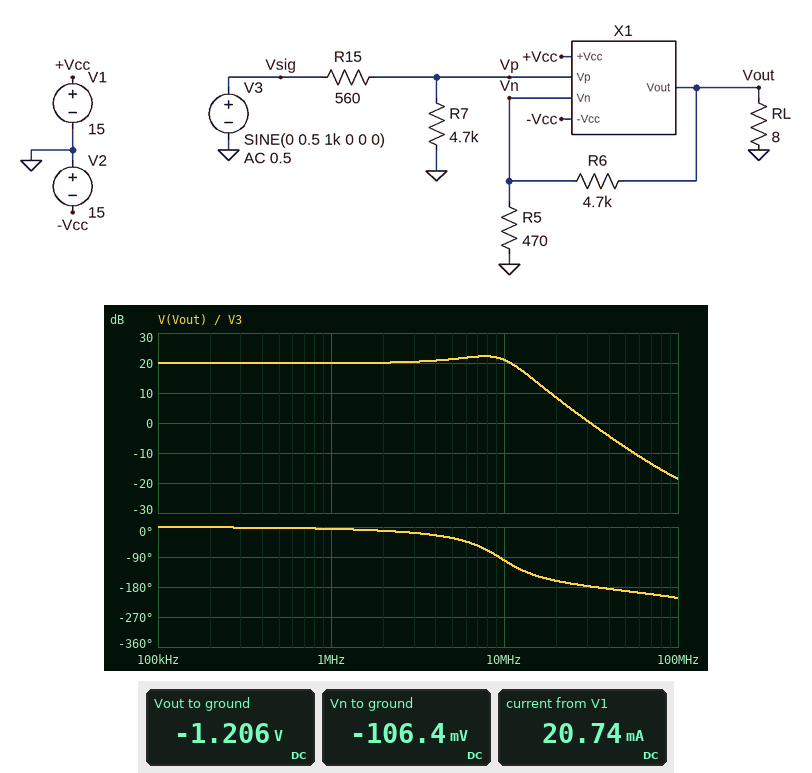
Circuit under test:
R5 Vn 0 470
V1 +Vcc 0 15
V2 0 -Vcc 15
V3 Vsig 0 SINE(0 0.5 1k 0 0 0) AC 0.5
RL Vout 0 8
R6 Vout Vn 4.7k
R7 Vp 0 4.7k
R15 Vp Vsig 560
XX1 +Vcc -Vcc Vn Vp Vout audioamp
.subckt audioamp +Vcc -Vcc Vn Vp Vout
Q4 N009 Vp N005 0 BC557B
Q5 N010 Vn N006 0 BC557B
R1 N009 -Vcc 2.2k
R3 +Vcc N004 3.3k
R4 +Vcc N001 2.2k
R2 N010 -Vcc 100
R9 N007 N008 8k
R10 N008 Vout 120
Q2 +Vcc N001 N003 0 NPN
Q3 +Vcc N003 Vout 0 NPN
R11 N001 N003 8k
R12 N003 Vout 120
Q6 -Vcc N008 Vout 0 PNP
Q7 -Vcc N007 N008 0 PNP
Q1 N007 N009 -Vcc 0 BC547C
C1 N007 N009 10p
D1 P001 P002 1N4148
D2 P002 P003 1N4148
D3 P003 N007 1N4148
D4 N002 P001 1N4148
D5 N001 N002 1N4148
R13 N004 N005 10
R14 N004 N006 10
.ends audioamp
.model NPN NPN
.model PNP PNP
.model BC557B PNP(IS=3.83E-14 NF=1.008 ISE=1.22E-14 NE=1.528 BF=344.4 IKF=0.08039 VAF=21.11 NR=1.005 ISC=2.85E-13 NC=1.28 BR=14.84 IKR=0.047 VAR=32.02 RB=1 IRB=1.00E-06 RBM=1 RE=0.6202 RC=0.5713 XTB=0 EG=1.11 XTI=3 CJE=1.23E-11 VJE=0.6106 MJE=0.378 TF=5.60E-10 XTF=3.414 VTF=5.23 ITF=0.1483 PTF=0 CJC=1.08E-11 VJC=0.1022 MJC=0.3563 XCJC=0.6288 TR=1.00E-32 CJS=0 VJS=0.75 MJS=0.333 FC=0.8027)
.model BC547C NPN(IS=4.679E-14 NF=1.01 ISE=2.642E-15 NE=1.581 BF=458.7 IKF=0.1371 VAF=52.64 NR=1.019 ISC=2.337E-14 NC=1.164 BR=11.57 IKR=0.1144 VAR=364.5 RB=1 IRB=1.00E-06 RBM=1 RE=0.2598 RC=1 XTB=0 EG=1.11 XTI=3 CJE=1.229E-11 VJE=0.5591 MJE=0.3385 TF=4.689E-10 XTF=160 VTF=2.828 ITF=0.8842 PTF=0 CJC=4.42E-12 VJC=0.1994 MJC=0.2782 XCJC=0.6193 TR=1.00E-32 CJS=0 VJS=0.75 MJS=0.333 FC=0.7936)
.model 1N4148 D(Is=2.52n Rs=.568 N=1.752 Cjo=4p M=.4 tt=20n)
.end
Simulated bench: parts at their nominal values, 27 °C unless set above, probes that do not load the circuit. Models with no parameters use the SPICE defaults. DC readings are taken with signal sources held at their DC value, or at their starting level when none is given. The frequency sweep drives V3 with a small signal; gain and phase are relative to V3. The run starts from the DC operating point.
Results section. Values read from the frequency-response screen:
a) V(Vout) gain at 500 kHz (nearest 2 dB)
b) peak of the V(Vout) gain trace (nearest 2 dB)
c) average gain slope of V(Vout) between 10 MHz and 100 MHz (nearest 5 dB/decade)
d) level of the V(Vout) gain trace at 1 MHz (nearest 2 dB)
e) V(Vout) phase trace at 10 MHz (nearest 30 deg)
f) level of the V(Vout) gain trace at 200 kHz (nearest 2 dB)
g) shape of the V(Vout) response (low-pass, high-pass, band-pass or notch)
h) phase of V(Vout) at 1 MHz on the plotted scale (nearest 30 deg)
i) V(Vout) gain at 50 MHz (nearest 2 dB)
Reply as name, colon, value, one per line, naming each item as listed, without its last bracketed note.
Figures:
V(Vout) gain at 500 kHz: 20 dB
peak of the V(Vout) gain trace: 22 dB
average gain slope of V(Vout) between 10 MHz and 100 MHz: -40 dB/decade
level of the V(Vout) gain trace at 1 MHz: 20 dB
V(Vout) phase trace at 10 MHz: -90 deg
level of the V(Vout) gain trace at 200 kHz: 20 dB
shape of the V(Vout) response: low-pass
phase of V(Vout) at 1 MHz on the plotted scale: 0 deg
V(Vout) gain at 50 MHz: -8 dB
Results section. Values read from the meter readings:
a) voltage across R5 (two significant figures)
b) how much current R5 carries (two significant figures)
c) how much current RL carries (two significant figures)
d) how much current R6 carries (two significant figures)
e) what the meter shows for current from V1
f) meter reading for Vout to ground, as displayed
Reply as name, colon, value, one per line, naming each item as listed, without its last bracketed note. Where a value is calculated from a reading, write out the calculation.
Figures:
voltage across R5: 0 V - (-106.4 mV) = 110 mV
how much current R5 carries: (0 V - (-106.4 mV)) / 470 Ω = 230 µA
how much current RL carries: (0 V - (-1.206 V)) / 8 Ω = 150 mA
how much current R6 carries: (-106.4 mV - (-1.206 V)) / 4.7 kΩ = 230 µA
what the meter shows for current from V1: 20.74 mA
meter reading for Vout to ground, as displayed: -1.206 V
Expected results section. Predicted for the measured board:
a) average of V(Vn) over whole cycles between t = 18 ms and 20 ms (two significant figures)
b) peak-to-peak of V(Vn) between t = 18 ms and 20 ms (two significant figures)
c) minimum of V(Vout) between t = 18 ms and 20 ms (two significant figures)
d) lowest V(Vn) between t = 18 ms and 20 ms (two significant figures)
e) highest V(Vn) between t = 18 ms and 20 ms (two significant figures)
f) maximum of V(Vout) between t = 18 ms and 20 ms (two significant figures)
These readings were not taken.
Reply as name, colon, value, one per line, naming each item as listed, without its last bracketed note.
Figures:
average of V(Vn) over whole cycles between t = 18 ms and 20 ms: -110 mV
peak-to-peak of V(Vn) between t = 18 ms and 20 ms: 900 mV
minimum of V(Vout) between t = 18 ms and 20 ms: -6.1 V
lowest V(Vn) between t = 18 ms and 20 ms: -550 mV
highest V(Vn) between t = 18 ms and 20 ms: 340 mV
maximum of V(Vout) between t = 18 ms and 20 ms: 3.7 V
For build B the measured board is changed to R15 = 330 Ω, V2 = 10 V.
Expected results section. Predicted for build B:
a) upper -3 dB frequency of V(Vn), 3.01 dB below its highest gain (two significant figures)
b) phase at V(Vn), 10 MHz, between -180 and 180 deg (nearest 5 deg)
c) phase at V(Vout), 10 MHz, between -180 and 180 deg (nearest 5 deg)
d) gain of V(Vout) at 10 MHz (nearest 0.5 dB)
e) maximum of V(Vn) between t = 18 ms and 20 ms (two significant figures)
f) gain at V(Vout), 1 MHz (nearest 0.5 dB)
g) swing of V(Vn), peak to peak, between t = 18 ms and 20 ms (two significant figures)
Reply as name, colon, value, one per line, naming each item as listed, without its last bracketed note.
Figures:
upper -3 dB frequency of V(Vn), 3.01 dB below its highest gain: 11 MHz
phase at V(Vn), 10 MHz, between -180 and 180 deg: -90 deg
phase at V(Vout), 10 MHz, between -180 and 180 deg: -80 deg
gain of V(Vout) at 10 MHz: 21.5 dB
maximum of V(Vn) between t = 18 ms and 20 ms: 360 mV
gain at V(Vout), 1 MHz: 20.5 dB
swing of V(Vn), peak to peak, between t = 18 ms and 20 ms: 940 mV
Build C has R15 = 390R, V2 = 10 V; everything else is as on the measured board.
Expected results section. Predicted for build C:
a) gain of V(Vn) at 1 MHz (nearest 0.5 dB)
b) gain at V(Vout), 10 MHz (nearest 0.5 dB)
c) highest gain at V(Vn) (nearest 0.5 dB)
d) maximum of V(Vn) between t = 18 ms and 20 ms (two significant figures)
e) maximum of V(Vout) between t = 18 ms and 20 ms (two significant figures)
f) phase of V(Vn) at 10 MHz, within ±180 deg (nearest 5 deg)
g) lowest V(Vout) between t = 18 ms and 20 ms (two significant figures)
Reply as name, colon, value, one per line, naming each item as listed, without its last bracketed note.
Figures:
gain of V(Vn) at 1 MHz: -0.5 dB
gain at V(Vout), 10 MHz: 21.5 dB
highest gain at V(Vn): 0 dB
maximum of V(Vn) between t = 18 ms and 20 ms: 360 mV
maximum of V(Vout) between t = 18 ms and 20 ms: 3.9 V
phase of V(Vn) at 10 MHz, within ±180 deg: -95 deg
lowest V(Vout) between t = 18 ms and 20 ms: -6.3 V
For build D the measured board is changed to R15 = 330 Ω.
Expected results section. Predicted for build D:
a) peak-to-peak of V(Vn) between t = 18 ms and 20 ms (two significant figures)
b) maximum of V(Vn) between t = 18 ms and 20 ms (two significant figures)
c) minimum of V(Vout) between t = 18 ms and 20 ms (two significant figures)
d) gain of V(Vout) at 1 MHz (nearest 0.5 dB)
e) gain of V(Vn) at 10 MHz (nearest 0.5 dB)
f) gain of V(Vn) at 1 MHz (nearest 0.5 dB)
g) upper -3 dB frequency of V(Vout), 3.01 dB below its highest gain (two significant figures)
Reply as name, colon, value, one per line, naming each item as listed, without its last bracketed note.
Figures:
peak-to-peak of V(Vn) between t = 18 ms and 20 ms: 940 mV
maximum of V(Vn) between t = 18 ms and 20 ms: 360 mV
minimum of V(Vout) between t = 18 ms and 20 ms: -6.4 V
gain of V(Vout) at 1 MHz: 20.5 dB
gain of V(Vn) at 10 MHz: -1.5 dB
gain of V(Vn) at 1 MHz: -0.5 dB
upper -3 dB frequency of V(Vout), 3.01 dB below its highest gain: 13 MHz
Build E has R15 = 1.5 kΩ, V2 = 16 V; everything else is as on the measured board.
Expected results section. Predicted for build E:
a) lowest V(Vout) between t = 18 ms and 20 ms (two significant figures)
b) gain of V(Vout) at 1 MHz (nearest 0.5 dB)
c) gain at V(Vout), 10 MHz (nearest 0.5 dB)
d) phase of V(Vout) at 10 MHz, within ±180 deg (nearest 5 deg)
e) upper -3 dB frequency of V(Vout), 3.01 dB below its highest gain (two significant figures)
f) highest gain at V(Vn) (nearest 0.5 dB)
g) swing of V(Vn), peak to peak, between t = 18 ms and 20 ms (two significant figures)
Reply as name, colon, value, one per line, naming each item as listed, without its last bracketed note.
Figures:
lowest V(Vout) between t = 18 ms and 20 ms: -5.4 V
gain of V(Vout) at 1 MHz: 18.5 dB
gain at V(Vout), 10 MHz: 15.0 dB
phase of V(Vout) at 10 MHz, within ±180 deg: -145 deg
upper -3 dB frequency of V(Vout), 3.01 dB below its highest gain: 8.1 MHz
highest gain at V(Vn): 1.0 dB
swing of V(Vn), peak to peak, between t = 18 ms and 20 ms: 760 mV
